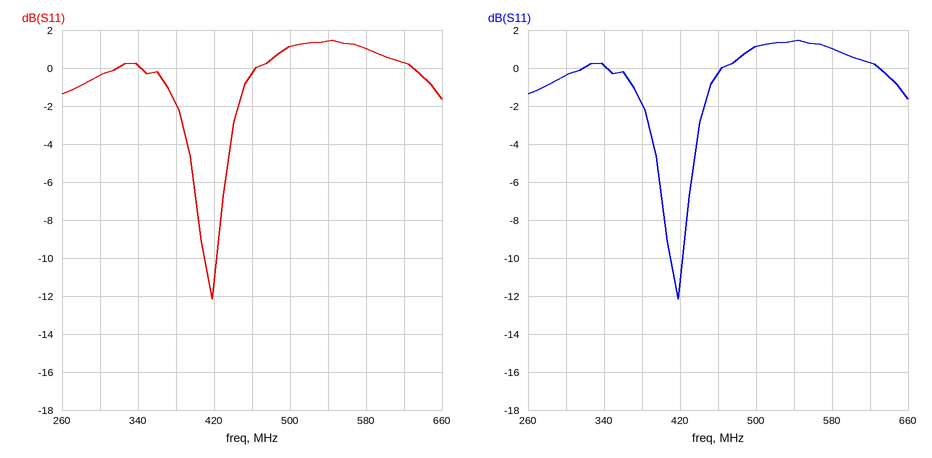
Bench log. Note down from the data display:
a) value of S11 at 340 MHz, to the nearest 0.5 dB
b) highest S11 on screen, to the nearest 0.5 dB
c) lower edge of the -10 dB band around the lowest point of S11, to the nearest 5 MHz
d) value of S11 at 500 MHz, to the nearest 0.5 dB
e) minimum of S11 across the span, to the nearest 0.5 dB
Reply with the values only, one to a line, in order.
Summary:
0.0 dB
1.5 dB
410 MHz
1.0 dB
-12.0 dB
